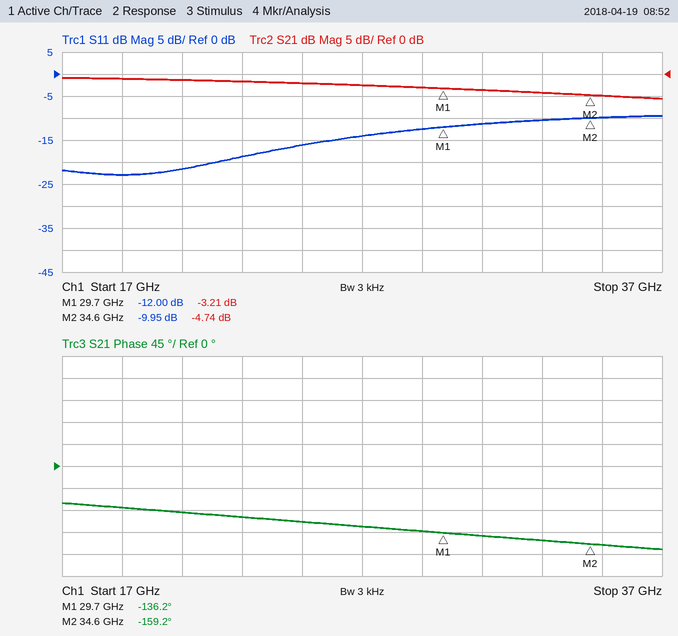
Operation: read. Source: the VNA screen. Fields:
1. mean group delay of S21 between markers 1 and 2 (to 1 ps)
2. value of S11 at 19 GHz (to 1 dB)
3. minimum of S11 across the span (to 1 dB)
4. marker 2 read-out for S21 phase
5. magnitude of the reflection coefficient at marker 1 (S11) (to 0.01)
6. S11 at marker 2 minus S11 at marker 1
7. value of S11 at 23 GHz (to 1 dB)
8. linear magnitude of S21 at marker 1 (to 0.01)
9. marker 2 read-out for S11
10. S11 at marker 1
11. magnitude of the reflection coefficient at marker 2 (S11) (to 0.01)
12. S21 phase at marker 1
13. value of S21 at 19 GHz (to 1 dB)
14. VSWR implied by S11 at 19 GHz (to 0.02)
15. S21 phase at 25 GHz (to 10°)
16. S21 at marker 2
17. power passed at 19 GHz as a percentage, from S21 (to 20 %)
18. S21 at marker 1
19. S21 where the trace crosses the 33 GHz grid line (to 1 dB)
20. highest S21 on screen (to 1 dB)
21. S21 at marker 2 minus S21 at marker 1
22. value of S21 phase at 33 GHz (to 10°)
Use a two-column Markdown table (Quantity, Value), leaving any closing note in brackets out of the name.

| Quantity | Value |
|---|---|
| mean group delay of S21 between markers 1 and 2 | 13 ps |
| value of S11 at 19 GHz | -23 dB |
| minimum of S11 across the span | -23 dB |
| marker 2 read-out for S21 phase | -159.2° |
| magnitude of the reflection coefficient at marker 1 (S11) | 0.25 |
| S11 at marker 2 minus S11 at marker 1 | 2.05 dB |
| value of S11 at 23 GHz | -19 dB |
| linear magnitude of S21 at marker 1 | 0.69 |
| marker 2 read-out for S11 | -9.95 dB |
| S11 at marker 1 | -12.00 dB |
| magnitude of the reflection coefficient at marker 2 (S11) | 0.32 |
| S21 phase at marker 1 | -136.2° |
| value of S21 at 19 GHz | -1 dB |
| VSWR implied by S11 at 19 GHz | 1.16 |
| S21 phase at 25 GHz | -110° |
| S21 at marker 2 | -4.74 dB |
| power passed at 19 GHz as a percentage, from S21 | 80 % |
| S21 at marker 1 | -3.21 dB |
| S21 where the trace crosses the 33 GHz grid line | -4 dB |
| highest S21 on screen | -1 dB |
| S21 at marker 2 minus S21 at marker 1 | -1.53 dB |
| value of S21 phase at 33 GHz | -150° |
